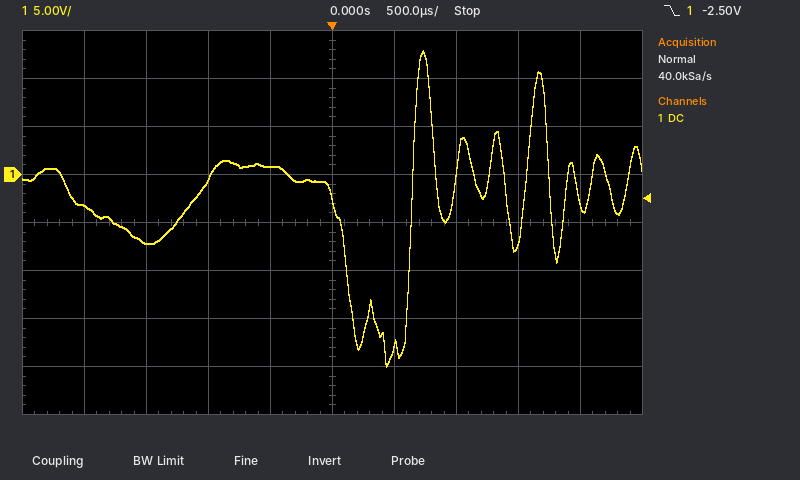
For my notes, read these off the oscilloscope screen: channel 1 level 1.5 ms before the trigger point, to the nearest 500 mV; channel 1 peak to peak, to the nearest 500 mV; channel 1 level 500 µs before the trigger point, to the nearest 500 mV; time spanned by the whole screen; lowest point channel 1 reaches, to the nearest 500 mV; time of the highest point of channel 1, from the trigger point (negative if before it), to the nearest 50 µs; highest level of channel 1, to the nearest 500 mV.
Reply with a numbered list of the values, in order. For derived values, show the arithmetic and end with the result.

1. -7.0 V
2. 13.0 V − (-20.0 V) = 33.0 V
3. 1.0 V
4. 5 ms
5. -20.0 V
6. +750 µs
7. 13.0 V
